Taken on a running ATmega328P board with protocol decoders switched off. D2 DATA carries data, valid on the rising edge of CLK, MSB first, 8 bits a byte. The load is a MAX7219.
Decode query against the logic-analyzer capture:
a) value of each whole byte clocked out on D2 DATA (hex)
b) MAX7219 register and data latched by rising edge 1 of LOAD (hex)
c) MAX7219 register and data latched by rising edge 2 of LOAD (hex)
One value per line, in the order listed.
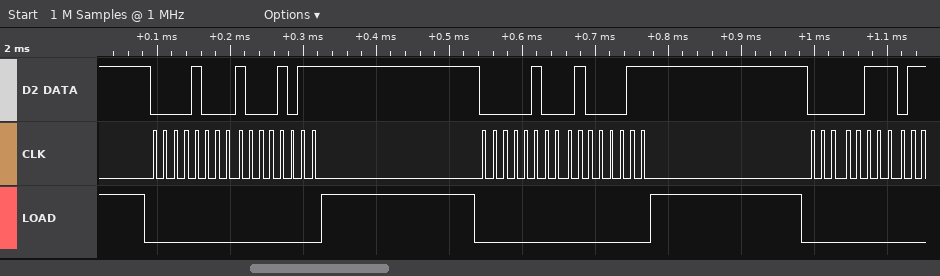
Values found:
08 8B 04 43 07
register 0x8, data 0x8B
register 0x4, data 0x43
